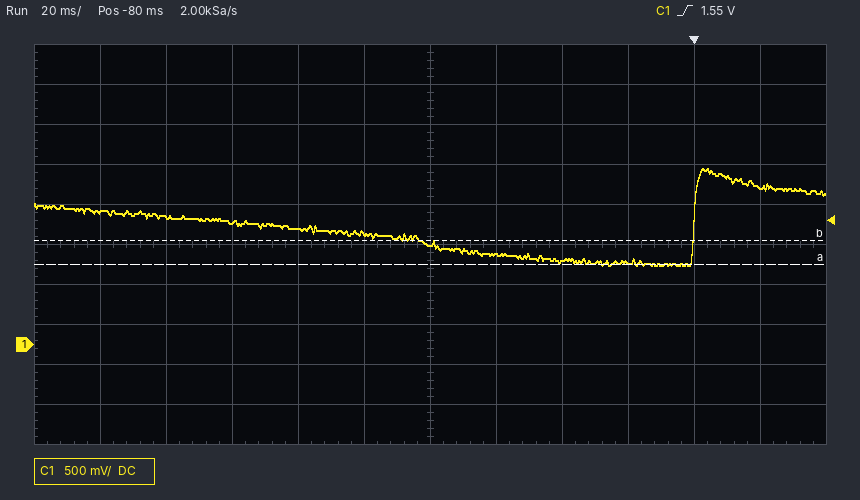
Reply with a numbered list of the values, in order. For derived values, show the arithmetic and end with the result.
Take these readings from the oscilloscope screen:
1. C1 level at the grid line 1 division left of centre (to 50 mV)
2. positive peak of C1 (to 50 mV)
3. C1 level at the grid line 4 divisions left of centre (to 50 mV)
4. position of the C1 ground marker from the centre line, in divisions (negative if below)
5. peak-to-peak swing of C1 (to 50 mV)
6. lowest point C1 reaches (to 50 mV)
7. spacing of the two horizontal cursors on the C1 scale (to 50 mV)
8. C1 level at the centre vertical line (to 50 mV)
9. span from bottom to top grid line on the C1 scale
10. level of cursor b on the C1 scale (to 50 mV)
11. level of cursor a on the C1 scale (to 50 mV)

1. 1.40 V
2. 2.20 V
3. 1.60 V
4. -2.5 div
5. 2.20 V − (1.00 V) = 1.20 V
6. 1.00 V
7. 300 mV
8. 1.25 V
9. 5 V
10. 1.30 V
11. 1.00 V
